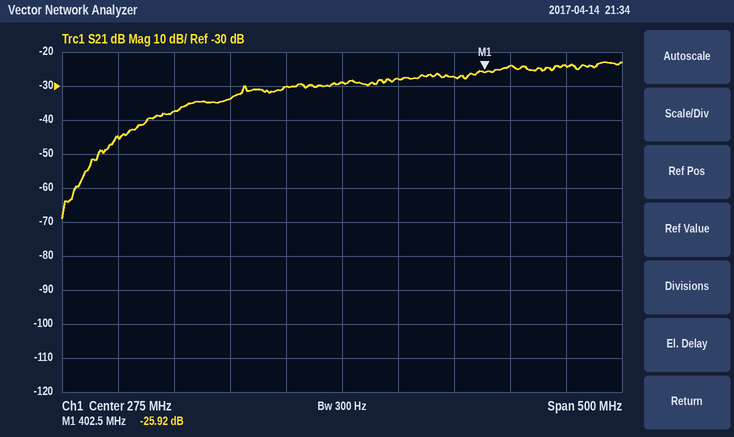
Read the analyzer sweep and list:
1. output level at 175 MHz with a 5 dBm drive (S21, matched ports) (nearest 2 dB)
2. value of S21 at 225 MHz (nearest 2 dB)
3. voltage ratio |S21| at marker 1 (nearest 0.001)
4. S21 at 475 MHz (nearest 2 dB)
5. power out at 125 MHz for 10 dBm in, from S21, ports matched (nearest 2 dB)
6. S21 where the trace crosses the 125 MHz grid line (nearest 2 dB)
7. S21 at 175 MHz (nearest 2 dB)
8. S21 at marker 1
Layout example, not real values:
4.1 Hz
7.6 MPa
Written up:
-28 dBm
-30 dB
0.051
-24 dB
-28 dBm
-38 dB
-34 dB
-25.92 dB
